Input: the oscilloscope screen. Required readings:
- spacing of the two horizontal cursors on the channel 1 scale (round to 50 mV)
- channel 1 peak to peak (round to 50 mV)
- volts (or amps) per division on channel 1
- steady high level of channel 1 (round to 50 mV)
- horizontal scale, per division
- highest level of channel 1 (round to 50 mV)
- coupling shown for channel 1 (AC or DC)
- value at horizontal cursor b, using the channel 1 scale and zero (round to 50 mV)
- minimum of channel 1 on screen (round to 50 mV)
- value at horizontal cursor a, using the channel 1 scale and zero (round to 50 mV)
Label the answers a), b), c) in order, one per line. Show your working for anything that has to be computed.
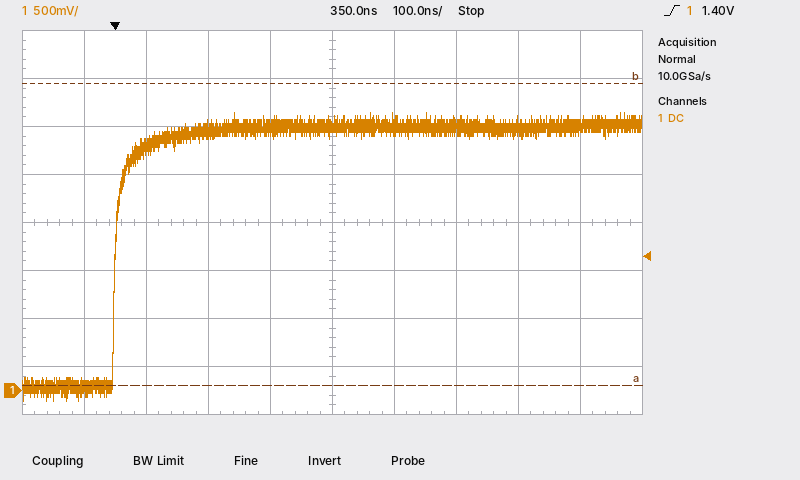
a) 3.15 V
b) 2.90 V − (-100 mV) = 3.00 V
c) 500 mV
d) 2.75 V
e) 100 ns
f) 2.90 V
g) DC
h) 3.20 V
i) -100 mV
j) 50 mV
